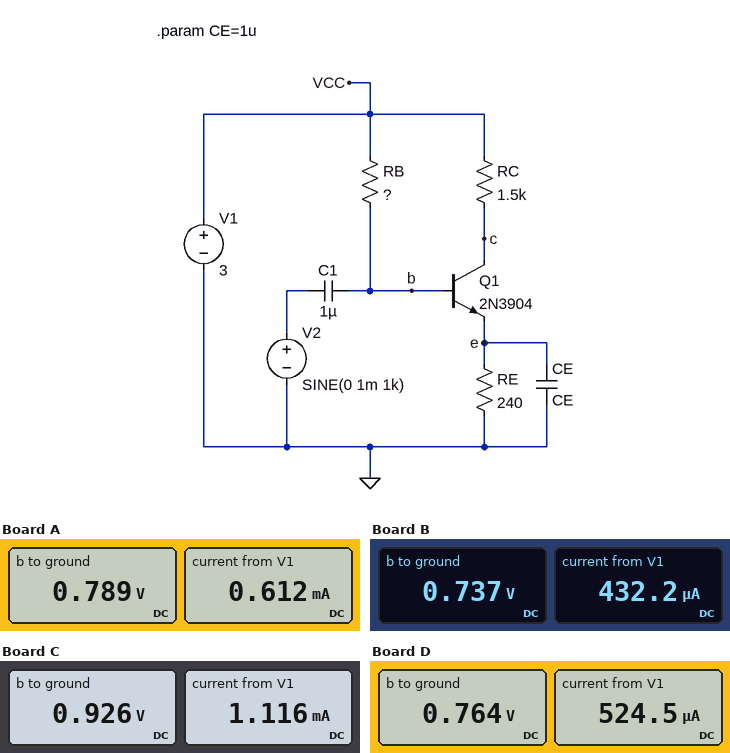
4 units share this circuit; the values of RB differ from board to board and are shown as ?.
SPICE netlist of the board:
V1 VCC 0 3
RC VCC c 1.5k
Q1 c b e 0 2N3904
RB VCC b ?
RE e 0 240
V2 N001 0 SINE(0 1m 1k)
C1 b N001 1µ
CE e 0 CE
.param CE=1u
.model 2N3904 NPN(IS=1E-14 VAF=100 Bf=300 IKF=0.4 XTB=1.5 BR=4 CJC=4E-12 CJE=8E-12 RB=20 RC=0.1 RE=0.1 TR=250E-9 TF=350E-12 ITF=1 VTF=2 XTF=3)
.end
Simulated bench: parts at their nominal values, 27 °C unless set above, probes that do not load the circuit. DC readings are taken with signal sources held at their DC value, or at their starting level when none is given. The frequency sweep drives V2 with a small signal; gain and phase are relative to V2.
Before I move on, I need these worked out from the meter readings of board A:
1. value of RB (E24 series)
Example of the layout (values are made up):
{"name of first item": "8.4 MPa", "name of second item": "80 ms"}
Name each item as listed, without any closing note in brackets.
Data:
{"value of RB": "1.1 MΩ"}
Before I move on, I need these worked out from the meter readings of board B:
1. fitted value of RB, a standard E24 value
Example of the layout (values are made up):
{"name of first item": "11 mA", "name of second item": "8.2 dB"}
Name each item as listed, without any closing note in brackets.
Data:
{"fitted value of RB, a standard E24 value": "1.6 MΩ"}
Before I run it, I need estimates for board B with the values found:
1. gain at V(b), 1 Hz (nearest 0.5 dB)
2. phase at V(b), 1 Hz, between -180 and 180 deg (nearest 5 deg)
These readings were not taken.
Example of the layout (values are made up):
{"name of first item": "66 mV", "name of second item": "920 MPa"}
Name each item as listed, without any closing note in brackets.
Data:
{"gain at V(b), 1 Hz": "-6.5 dB", "phase at V(b), 1 Hz, between -180 and 180 deg": "60 deg"}
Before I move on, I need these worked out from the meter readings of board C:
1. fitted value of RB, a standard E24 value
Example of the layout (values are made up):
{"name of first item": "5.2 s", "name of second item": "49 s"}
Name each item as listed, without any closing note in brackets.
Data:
{"fitted value of RB, a standard E24 value": "560 kΩ"}
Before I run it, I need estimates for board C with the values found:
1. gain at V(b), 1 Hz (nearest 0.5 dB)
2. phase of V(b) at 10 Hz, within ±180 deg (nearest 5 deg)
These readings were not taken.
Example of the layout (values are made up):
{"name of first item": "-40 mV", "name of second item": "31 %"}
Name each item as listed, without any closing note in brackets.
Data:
{"gain at V(b), 1 Hz": "-8.0 dB", "phase of V(b) at 10 Hz, within ±180 deg": "15 deg"}
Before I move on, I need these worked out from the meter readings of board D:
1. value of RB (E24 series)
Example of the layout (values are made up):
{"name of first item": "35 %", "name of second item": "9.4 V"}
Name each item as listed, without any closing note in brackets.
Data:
{"value of RB": "1.3 MΩ"}
